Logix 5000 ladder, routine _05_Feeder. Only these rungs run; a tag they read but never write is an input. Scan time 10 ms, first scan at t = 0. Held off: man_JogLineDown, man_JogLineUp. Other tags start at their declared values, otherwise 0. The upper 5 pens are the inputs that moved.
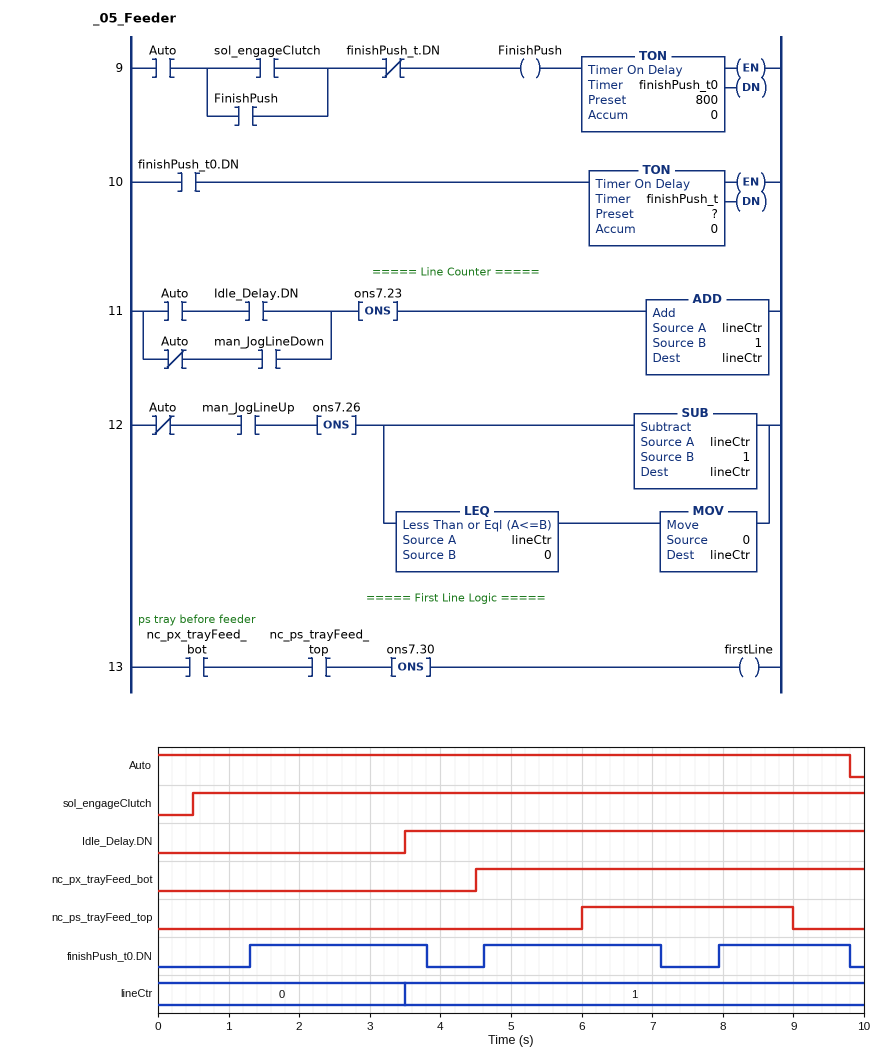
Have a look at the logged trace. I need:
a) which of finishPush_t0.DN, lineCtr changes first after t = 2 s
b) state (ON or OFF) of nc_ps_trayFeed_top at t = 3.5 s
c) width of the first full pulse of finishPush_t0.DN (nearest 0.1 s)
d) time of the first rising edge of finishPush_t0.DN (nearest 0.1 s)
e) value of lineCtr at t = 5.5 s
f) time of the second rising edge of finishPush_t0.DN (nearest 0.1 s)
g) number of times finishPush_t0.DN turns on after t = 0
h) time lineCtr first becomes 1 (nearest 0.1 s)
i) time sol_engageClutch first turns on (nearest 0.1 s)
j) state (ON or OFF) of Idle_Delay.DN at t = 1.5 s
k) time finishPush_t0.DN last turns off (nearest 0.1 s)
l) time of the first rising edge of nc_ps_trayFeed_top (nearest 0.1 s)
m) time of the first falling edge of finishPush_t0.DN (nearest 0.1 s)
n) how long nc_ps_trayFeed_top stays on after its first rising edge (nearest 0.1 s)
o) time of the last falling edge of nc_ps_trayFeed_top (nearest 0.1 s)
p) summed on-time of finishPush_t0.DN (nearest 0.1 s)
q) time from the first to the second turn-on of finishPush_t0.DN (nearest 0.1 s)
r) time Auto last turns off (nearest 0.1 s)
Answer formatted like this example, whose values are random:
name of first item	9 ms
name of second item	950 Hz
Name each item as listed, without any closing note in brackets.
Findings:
which of finishPush_t0.DN, lineCtr changes first after t = 2 s	lineCtr
state (ON or OFF) of nc_ps_trayFeed_top at t = 3.5 s	OFF
width of the first full pulse of finishPush_t0.DN	2.5 s
time of the first rising edge of finishPush_t0.DN	1.3 s
value of lineCtr at t = 5.5 s	1
time of the second rising edge of finishPush_t0.DN	4.6 s
number of times finishPush_t0.DN turns on after t = 0	3
time lineCtr first becomes 1	3.5 s
time sol_engageClutch first turns on	0.5 s
state (ON or OFF) of Idle_Delay.DN at t = 1.5 s	OFF
time finishPush_t0.DN last turns off	9.8 s
time of the first rising edge of nc_ps_trayFeed_top	6.0 s
time of the first falling edge of finishPush_t0.DN	3.8 s
how long nc_ps_trayFeed_top stays on after its first rising edge	3.0 s
time of the last falling edge of nc_ps_trayFeed_top	9.0 s
summed on-time of finishPush_t0.DN	6.9 s
time from the first to the second turn-on of finishPush_t0.DN	3.3 s
time Auto last turns off	9.8 s
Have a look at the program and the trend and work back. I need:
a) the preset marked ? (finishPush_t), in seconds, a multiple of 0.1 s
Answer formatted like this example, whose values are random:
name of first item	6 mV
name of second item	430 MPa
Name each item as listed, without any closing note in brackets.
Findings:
the preset marked ? (finishPush_t), in seconds, a multiple of 0.1 s	2.5 s
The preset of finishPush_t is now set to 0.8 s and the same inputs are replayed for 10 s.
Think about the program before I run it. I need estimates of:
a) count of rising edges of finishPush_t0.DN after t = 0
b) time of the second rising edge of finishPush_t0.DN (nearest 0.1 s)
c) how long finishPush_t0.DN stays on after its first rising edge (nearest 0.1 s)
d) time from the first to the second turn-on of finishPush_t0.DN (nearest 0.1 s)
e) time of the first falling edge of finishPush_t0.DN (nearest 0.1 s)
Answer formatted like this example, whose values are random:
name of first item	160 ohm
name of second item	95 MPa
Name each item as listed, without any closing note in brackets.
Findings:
count of rising edges of finishPush_t0.DN after t = 0	6
time of the second rising edge of finishPush_t0.DN	2.9 s
how long finishPush_t0.DN stays on after its first rising edge	0.8 s
time from the first to the second turn-on of finishPush_t0.DN	1.6 s
time of the first falling edge of finishPush_t0.DN	2.1 s
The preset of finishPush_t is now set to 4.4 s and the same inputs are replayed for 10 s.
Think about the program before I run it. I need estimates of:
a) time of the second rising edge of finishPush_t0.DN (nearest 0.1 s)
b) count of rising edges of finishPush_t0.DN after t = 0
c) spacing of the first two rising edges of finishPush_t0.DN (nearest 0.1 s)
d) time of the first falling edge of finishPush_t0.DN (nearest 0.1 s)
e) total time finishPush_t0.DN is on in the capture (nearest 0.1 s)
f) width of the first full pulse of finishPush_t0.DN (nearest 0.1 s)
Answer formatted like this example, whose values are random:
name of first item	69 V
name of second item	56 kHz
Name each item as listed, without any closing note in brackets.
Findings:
time of the second rising edge of finishPush_t0.DN	6.5 s
count of rising edges of finishPush_t0.DN after t = 0	2
spacing of the first two rising edges of finishPush_t0.DN	5.2 s
time of the first falling edge of finishPush_t0.DN	5.7 s
total time finishPush_t0.DN is on in the capture	7.7 s
width of the first full pulse of finishPush_t0.DN	4.4 s
